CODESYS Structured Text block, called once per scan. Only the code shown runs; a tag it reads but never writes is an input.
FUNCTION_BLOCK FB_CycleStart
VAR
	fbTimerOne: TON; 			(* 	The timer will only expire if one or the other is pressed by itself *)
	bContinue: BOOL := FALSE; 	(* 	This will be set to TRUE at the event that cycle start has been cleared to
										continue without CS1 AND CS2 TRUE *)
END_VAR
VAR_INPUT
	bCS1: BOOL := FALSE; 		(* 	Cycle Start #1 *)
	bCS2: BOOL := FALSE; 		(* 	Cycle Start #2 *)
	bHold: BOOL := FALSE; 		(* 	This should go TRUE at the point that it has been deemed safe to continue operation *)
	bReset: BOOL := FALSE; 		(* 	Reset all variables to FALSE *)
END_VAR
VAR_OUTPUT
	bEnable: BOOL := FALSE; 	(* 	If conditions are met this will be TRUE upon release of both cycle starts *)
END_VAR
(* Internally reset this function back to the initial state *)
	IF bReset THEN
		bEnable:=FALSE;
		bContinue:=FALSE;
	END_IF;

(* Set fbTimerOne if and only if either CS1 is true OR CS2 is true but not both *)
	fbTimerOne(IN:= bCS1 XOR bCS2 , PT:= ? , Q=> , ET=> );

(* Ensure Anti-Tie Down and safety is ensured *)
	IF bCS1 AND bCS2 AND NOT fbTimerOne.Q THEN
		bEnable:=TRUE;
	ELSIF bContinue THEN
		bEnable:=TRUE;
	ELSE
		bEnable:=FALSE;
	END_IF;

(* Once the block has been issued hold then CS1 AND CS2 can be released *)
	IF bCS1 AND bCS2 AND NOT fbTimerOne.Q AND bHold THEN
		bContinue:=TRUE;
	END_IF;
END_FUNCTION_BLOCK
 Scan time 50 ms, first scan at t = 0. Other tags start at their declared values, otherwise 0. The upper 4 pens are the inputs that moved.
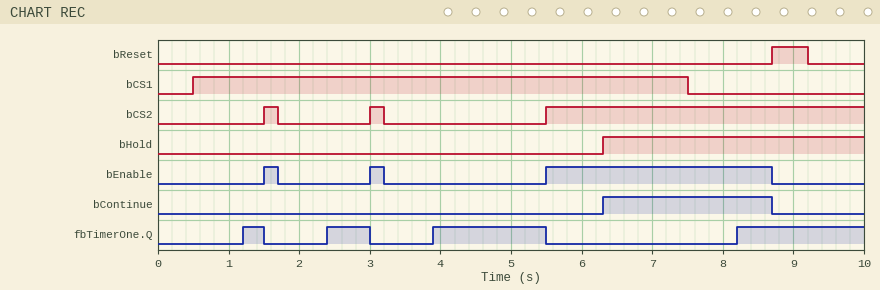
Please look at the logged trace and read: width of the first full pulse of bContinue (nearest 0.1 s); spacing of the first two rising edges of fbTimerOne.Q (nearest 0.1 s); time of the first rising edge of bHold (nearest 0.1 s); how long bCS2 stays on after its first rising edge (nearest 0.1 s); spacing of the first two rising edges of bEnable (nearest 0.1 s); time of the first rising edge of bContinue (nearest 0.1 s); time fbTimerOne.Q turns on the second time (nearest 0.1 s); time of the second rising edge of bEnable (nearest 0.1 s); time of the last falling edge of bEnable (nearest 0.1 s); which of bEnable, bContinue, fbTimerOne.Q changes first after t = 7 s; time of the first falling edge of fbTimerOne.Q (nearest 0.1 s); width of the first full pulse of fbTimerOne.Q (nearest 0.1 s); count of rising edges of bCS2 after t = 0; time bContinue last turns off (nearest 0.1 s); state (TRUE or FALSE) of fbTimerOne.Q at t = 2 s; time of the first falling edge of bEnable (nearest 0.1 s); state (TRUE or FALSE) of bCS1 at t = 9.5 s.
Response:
2.4 s
1.2 s
6.3 s
0.2 s
1.5 s
6.3 s
2.4 s
3.0 s
8.7 s
fbTimerOne.Q
1.5 s
0.3 s
3
8.7 s
FALSE
1.7 s
FALSE
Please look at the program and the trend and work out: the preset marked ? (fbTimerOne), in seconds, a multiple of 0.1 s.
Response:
0.7 s
